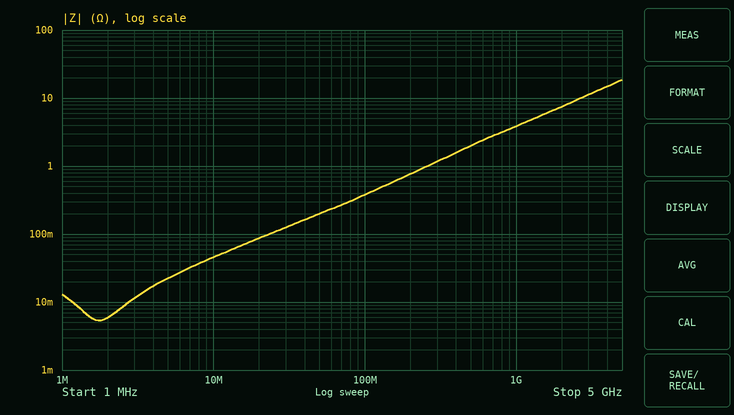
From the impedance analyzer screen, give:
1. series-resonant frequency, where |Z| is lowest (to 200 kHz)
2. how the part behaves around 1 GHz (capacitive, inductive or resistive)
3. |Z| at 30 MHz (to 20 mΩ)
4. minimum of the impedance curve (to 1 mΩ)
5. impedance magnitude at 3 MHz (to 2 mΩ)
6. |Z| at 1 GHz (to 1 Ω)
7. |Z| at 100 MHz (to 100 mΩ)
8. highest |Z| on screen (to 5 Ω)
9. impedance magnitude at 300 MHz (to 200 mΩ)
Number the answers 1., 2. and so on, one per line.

1. 1.8 MHz
2. inductive
3. 120 mΩ
4. 5 mΩ
5. 12 mΩ
6. 4 Ω
7. 400 mΩ
8. 20 Ω
9. 1.2 Ω
